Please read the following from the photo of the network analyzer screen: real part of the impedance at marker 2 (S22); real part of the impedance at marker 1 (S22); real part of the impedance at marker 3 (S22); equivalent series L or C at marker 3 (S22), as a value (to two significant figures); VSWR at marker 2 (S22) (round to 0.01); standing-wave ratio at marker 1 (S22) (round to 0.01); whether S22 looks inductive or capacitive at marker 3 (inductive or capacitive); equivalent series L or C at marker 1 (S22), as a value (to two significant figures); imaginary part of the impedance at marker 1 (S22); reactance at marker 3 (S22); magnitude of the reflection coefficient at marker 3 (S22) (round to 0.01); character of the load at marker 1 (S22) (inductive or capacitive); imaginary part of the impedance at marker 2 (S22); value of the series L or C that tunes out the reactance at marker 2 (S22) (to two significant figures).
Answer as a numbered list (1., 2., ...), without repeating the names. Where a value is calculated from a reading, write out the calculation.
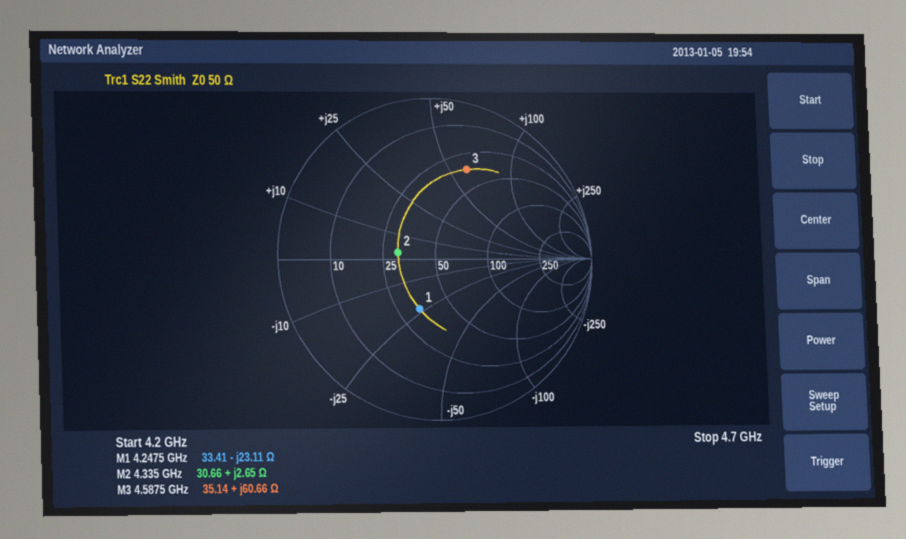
1. 30.66 Ω
2. 33.41 Ω
3. 35.14 Ω
4. L = 60.66 Ω/(2π × 4.5875 GHz) ≈ 2.1 nH
5. 1.64
6. 1.98
7. inductive
8. C = 1/(2π × 4.2475 GHz × 23.11 Ω) ≈ 1.6 pF
9. -23.11 Ω
10. +60.66 Ω
11. 0.60
12. capacitive
13. +2.65 Ω
14. C = 1/(2π × 4.335 GHz × 2.65 Ω) ≈ 14 pF
